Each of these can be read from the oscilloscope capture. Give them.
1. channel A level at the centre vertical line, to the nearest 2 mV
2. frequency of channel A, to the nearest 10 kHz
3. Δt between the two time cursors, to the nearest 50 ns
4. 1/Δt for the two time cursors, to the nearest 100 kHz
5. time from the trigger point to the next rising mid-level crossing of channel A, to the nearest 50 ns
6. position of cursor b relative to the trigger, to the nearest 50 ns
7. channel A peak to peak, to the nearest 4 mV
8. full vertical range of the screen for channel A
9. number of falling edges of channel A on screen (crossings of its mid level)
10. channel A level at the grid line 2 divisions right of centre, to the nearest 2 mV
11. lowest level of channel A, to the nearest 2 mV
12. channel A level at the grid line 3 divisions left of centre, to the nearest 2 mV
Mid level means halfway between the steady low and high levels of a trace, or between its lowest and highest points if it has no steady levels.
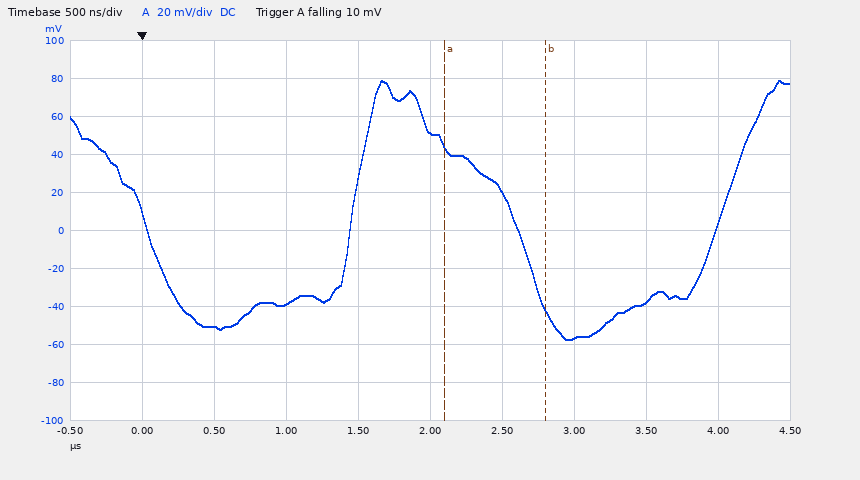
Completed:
52 mV
390 kHz
700 ns
1.4 MHz
1.45 µs
+2.80 µs
136 mV
200 mV
2
-56 mV
-58 mV
-50 mV
